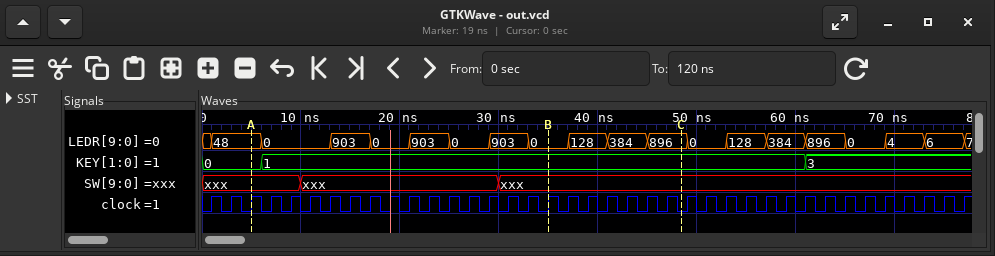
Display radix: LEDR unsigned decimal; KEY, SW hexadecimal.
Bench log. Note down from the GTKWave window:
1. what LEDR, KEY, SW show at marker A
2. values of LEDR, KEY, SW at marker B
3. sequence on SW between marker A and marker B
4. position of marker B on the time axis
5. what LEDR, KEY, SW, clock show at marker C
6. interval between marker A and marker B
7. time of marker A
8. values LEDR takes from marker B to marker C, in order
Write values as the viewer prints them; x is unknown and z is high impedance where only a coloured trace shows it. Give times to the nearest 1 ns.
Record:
LEDR=48, KEY=0, SW=xxx
LEDR=0, KEY=1, SW=xxx
xxx, xxx, xxx
35 ns
LEDR=896, KEY=1, SW=xxx, clock=0
30 ns
5 ns
0, 128, 384, 896
